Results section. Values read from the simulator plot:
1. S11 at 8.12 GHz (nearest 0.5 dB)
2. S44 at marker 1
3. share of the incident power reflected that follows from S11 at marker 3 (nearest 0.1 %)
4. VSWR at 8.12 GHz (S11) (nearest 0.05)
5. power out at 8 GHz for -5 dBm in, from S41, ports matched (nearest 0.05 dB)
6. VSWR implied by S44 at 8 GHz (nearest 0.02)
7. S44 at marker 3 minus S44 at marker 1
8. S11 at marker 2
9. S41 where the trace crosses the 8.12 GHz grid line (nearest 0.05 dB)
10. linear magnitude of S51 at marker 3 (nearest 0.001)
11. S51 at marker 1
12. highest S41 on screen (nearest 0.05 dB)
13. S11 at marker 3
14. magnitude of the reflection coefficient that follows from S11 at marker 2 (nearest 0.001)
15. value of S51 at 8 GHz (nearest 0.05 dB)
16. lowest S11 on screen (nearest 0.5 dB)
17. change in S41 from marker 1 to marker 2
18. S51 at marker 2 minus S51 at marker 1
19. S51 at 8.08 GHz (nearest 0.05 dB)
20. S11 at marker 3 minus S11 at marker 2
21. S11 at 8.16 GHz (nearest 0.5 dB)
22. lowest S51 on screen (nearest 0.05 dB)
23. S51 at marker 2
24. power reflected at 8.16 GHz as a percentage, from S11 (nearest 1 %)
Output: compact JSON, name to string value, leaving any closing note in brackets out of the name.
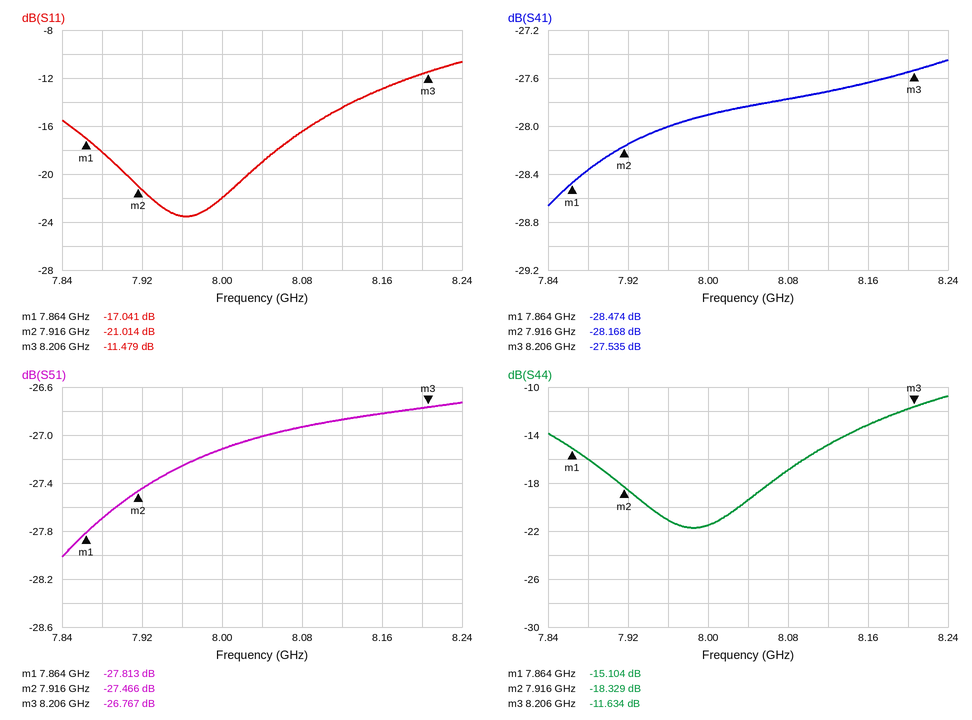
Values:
{"S11 at 8.12 GHz": "-14.5 dB", "S44 at marker 1": "-15.104 dB", "share of the incident power reflected that follows from S11 at marker 3": "7.1 %", "VSWR at 8.12 GHz (S11)": "1.45", "power out at 8 GHz for -5 dBm in, from S41, ports matched": "-32.90 dBm", "VSWR implied by S44 at 8 GHz": "1.18", "S44 at marker 3 minus S44 at marker 1": "3.470 dB", "S11 at marker 2": "-21.014 dB", "S41 where the trace crosses the 8.12 GHz grid line": "-27.70 dB", "linear magnitude of S51 at marker 3": "0.046", "S51 at marker 1": "-27.813 dB", "highest S41 on screen": "-27.45 dB", "S11 at marker 3": "-11.479 dB", "magnitude of the reflection coefficient that follows from S11 at marker 2": "0.089", "value of S51 at 8 GHz": "-27.10 dB", "lowest S11 on screen": "-23.5 dB", "change in S41 from marker 1 to marker 2": "0.306 dB", "S51 at marker 2 minus S51 at marker 1": "0.347 dB", "S51 at 8.08 GHz": "-26.95 dB", "S11 at marker 3 minus S11 at marker 2": "9.535 dB", "S11 at 8.16 GHz": "-13.0 dB", "lowest S51 on screen": "-28.00 dB", "S51 at marker 2": "-27.466 dB", "power reflected at 8.16 GHz as a percentage, from S11": "5 %"}
